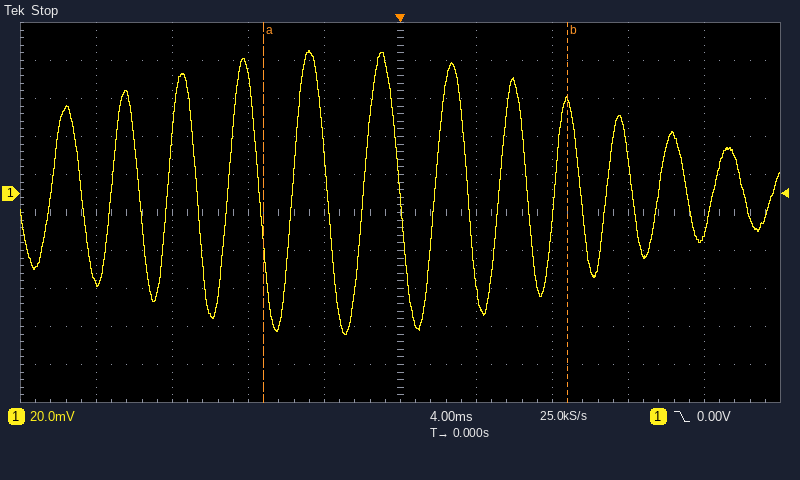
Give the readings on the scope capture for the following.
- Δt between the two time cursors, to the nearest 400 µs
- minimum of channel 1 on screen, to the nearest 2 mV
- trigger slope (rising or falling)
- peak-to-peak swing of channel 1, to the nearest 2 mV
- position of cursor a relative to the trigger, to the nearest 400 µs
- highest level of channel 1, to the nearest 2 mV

16.0 ms
-74 mV
falling
150 mV
-7.2 ms
76 mV
